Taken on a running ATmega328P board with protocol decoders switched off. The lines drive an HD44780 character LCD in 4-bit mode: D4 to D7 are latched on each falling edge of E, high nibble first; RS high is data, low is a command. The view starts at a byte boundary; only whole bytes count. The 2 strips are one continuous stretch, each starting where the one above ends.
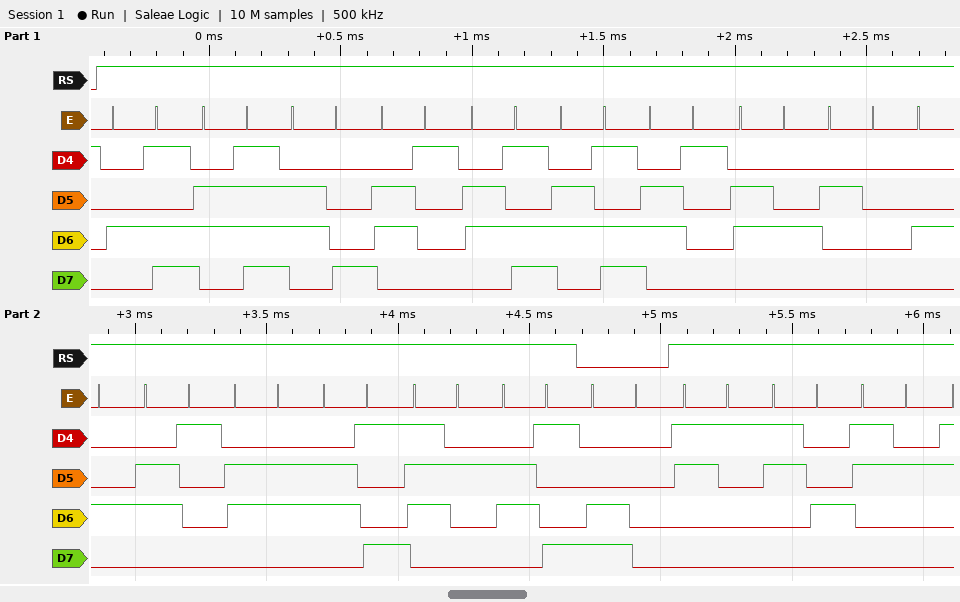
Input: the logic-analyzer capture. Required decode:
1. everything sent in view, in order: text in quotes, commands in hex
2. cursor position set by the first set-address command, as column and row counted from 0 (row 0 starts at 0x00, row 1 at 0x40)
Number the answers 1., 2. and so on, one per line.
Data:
1. "Mohammad Dafiri" 0xC0 "142"
2. column 0, row 1
